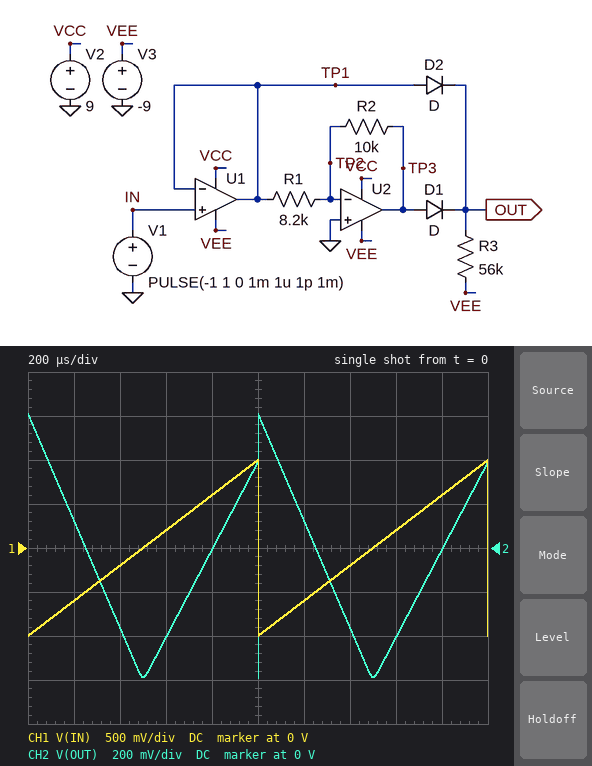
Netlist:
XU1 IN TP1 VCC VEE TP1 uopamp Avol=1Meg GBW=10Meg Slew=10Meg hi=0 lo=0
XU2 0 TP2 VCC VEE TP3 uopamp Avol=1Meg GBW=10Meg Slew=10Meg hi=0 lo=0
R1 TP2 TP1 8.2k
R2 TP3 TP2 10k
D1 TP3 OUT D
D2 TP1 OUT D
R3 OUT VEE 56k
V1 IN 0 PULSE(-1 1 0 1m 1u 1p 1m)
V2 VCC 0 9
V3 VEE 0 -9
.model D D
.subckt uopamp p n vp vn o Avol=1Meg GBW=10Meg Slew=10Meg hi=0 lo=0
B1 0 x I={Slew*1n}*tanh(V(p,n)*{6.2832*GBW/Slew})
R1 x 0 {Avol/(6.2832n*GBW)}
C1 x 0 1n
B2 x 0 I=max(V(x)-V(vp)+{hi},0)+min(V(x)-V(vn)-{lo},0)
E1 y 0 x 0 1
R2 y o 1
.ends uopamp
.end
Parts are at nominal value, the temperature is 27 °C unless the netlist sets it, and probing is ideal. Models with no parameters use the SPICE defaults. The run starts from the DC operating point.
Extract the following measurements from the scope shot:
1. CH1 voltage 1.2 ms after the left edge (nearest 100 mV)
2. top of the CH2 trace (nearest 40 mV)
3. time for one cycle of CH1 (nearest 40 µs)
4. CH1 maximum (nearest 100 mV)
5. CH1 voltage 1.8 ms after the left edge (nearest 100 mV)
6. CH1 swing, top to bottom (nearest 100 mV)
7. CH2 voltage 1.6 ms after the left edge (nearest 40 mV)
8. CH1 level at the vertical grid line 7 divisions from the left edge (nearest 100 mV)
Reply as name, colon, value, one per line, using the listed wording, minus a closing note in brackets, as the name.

CH1 voltage 1.2 ms after the left edge: -600 mV
top of the CH2 trace: 600 mV
time for one cycle of CH1: 1.00 ms
CH1 maximum: 1.0 V
CH1 voltage 1.8 ms after the left edge: 600 mV
CH1 swing, top to bottom: 2.0 V
CH2 voltage 1.6 ms after the left edge: -400 mV
CH1 level at the vertical grid line 7 divisions from the left edge: -200 mV
